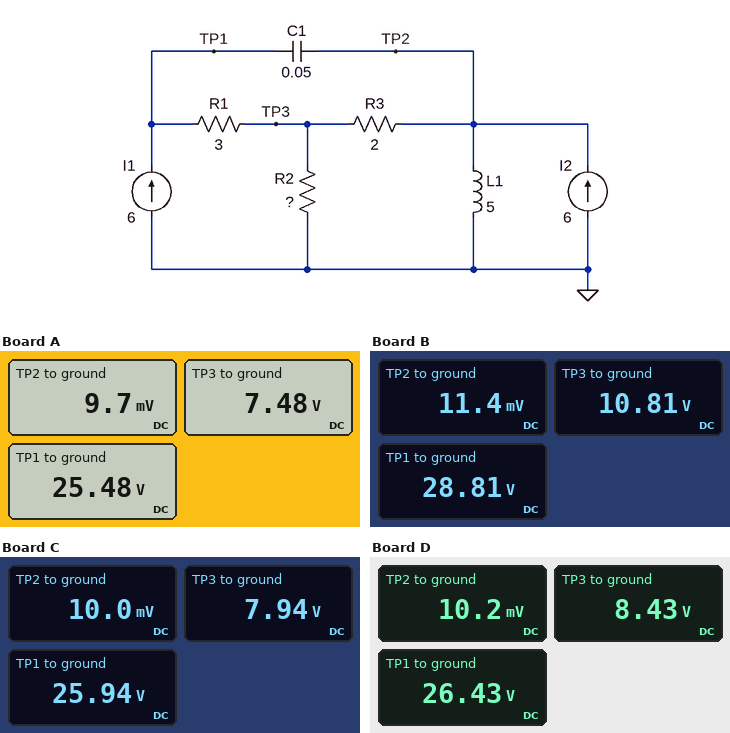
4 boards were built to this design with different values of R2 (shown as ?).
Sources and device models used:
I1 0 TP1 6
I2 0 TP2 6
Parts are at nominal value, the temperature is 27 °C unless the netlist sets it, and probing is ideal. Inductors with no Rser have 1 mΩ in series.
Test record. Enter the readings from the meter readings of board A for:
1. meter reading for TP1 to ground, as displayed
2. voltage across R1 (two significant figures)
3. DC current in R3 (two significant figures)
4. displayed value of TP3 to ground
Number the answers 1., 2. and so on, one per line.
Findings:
1. 25.48 V
2. 18 V
3. 3.7 A
4. 7.48 V
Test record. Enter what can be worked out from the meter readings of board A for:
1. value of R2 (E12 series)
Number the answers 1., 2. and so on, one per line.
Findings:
1. 3.3 Ω
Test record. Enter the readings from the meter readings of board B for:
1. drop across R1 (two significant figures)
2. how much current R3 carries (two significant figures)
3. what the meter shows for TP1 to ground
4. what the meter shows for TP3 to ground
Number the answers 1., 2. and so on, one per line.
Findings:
1. 18 V
2. 5.4 A
3. 28.81 V
4. 10.81 V
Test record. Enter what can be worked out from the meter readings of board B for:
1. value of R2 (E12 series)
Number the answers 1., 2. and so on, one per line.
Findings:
1. 18 Ω
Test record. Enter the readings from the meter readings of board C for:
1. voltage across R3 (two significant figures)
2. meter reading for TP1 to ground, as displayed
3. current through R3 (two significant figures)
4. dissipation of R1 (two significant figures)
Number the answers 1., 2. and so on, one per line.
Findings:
1. 7.9 V
2. 25.94 V
3. 4.0 A
4. 110 W
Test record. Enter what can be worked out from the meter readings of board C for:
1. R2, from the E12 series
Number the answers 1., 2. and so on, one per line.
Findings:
1. 3.9 Ω
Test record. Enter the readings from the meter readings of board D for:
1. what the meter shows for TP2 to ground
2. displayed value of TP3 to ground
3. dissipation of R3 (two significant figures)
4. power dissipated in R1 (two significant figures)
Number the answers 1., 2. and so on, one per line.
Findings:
1. 10.2 mV
2. 8.43 V
3. 35 W
4. 110 W
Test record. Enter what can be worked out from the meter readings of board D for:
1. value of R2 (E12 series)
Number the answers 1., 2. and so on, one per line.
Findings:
1. 4.7 Ω
